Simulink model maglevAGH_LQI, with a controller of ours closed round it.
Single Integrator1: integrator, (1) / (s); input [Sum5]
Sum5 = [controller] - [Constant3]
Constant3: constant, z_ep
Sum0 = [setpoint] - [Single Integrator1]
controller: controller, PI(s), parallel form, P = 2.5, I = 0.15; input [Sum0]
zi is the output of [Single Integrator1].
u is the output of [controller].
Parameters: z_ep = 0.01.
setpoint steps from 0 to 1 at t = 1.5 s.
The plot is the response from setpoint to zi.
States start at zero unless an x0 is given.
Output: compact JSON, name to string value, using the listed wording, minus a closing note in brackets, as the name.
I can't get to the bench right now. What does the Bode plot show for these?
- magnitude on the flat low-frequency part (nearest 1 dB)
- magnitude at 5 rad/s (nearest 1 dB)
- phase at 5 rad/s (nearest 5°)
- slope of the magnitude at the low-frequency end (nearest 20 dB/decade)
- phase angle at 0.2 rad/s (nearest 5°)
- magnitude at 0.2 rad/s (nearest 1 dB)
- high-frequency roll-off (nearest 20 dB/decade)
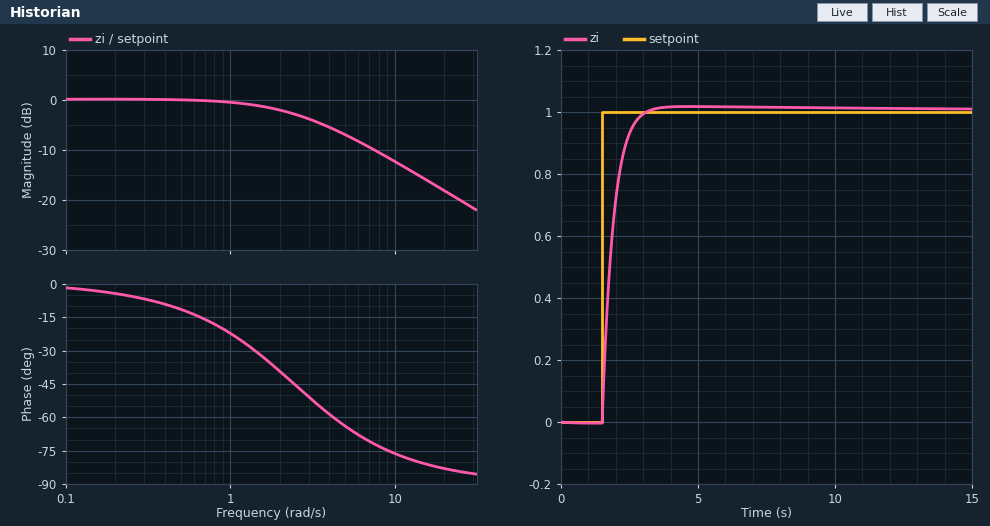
{"magnitude on the flat low-frequency part": "0 dB", "magnitude at 5 rad/s": "-7 dB", "phase at 5 rad/s": "-65°", "slope of the magnitude at the low-frequency end": "0 dB/decade", "phase angle at 0.2 rad/s": "-5°", "magnitude at 0.2 rad/s": "0 dB", "high-frequency roll-off": "-20 dB/decade"}
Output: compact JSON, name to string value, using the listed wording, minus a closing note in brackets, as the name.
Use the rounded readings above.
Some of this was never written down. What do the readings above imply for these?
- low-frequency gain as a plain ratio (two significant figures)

{"low-frequency gain as a plain ratio": "1.0"}
